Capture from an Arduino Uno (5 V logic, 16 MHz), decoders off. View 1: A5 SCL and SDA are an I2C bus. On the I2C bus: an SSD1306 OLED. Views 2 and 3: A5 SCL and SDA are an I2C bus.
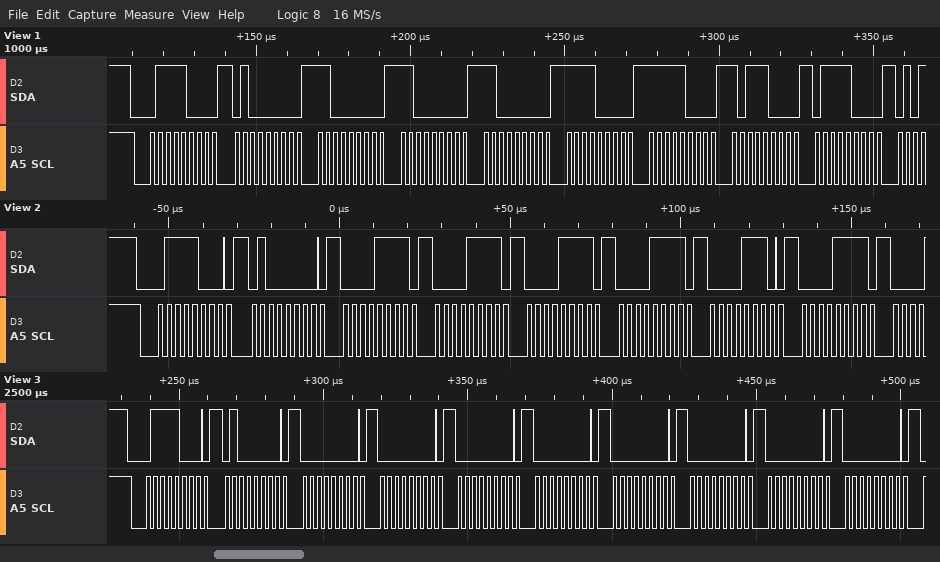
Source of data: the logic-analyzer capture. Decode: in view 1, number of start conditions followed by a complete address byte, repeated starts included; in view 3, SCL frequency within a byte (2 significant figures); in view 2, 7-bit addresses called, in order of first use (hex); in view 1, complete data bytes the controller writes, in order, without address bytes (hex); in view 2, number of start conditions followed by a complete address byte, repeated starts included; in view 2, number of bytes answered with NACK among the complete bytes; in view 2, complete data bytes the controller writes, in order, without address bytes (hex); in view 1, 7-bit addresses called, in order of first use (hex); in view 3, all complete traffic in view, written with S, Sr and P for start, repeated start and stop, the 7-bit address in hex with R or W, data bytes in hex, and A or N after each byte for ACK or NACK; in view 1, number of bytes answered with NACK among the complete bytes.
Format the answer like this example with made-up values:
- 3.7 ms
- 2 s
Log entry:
- 1
- 400 kHz
- 0x3C
- 40 C0 C0 C0 F0 F8 B8 78
- 1
- 0
- 40 0F 0F 0F 0F 0E 0F
- 0x3C
- S 3CW A 40 A 00 A 00 A 00 A 00 A 00 A 00 A 00 A 00 A
- 0
